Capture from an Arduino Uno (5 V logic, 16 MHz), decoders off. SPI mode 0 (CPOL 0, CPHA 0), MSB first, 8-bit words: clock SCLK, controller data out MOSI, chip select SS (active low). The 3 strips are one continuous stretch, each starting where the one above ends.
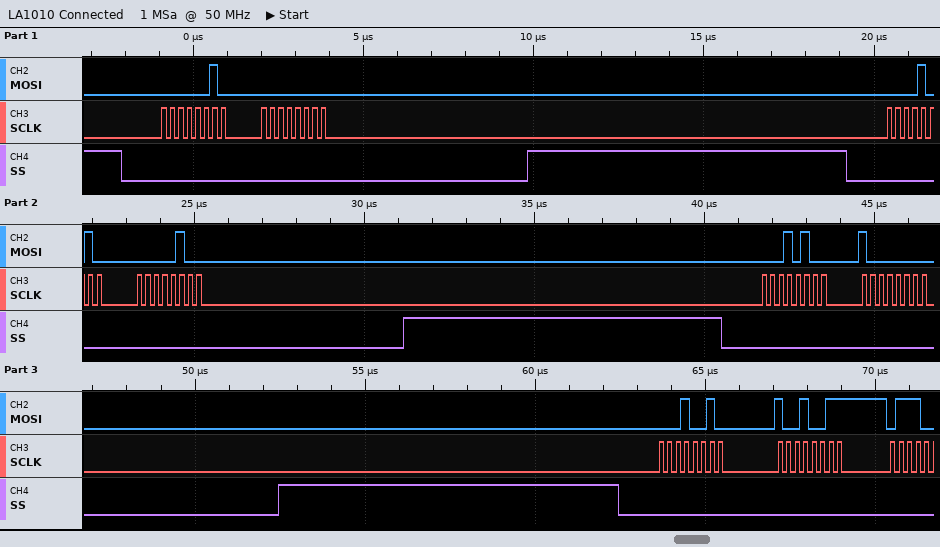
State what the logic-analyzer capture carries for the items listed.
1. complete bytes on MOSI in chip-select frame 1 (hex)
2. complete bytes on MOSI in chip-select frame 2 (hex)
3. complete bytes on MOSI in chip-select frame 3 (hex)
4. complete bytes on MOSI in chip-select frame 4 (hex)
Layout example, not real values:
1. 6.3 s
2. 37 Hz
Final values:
1. 02 00
2. 0A 04
3. 14 80
4. 12 93
